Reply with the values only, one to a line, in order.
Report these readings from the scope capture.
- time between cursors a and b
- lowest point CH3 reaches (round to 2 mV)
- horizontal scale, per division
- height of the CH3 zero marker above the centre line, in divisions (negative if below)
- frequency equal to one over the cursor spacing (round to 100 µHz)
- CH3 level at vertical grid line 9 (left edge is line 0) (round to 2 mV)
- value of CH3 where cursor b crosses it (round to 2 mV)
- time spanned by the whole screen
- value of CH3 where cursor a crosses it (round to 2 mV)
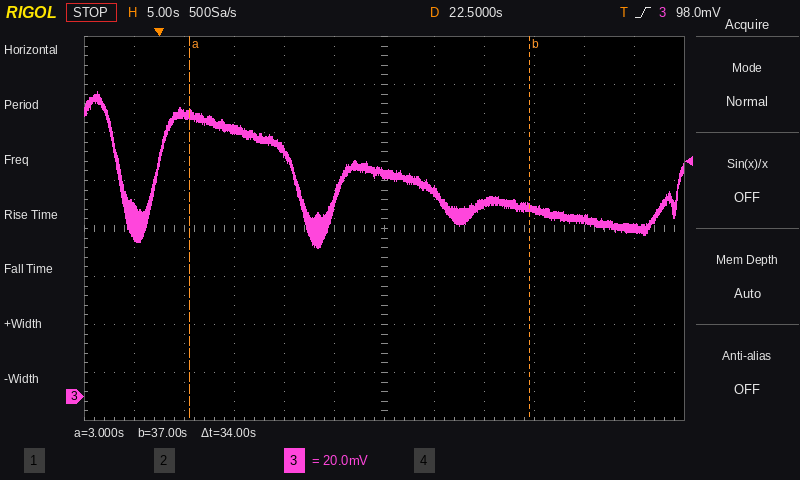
34 s
62 mV
5 s
-3.5 div
29.4 mHz
78 mV
78 mV
60 s
118 mV
